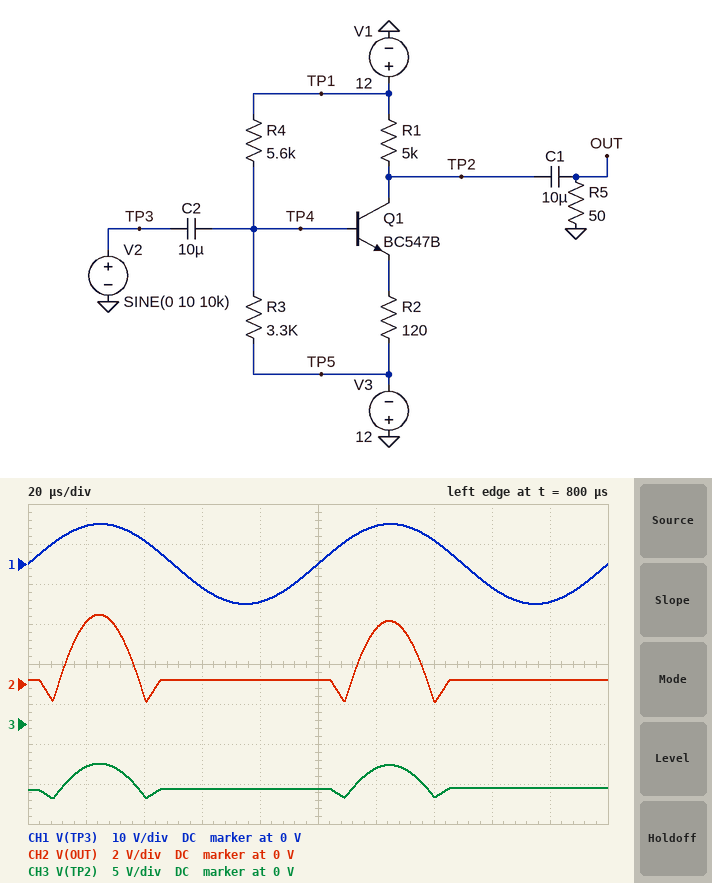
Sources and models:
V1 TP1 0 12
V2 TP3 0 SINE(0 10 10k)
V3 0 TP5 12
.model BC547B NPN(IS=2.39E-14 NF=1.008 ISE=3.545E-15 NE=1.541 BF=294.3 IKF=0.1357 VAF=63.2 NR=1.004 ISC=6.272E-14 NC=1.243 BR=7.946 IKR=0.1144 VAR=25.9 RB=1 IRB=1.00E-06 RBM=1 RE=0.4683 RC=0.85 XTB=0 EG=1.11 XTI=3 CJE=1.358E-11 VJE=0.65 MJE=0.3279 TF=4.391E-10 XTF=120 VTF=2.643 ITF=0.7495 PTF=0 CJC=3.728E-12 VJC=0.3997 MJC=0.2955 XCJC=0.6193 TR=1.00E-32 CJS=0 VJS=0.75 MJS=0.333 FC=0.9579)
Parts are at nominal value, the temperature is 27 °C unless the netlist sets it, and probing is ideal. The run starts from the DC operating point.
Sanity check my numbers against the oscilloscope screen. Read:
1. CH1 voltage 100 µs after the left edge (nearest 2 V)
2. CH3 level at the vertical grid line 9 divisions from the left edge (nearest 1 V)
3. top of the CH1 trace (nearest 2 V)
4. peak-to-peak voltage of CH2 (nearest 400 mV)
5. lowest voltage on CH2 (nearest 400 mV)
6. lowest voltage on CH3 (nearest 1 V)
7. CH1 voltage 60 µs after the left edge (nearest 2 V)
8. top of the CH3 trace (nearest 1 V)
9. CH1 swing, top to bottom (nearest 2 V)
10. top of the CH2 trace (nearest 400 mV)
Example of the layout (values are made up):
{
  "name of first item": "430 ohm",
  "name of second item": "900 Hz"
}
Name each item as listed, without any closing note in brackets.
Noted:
{
  "CH1 voltage 100 µs after the left edge": "0 V",
  "CH3 level at the vertical grid line 9 divisions from the left edge": "-8 V",
  "top of the CH1 trace": "10 V",
  "peak-to-peak voltage of CH2": "4.4 V",
  "lowest voltage on CH2": "-800 mV",
  "lowest voltage on CH3": "-9 V",
  "CH1 voltage 60 µs after the left edge": "-6 V",
  "top of the CH3 trace": "-5 V",
  "CH1 swing, top to bottom": "20 V",
  "top of the CH2 trace": "3.6 V"
}
